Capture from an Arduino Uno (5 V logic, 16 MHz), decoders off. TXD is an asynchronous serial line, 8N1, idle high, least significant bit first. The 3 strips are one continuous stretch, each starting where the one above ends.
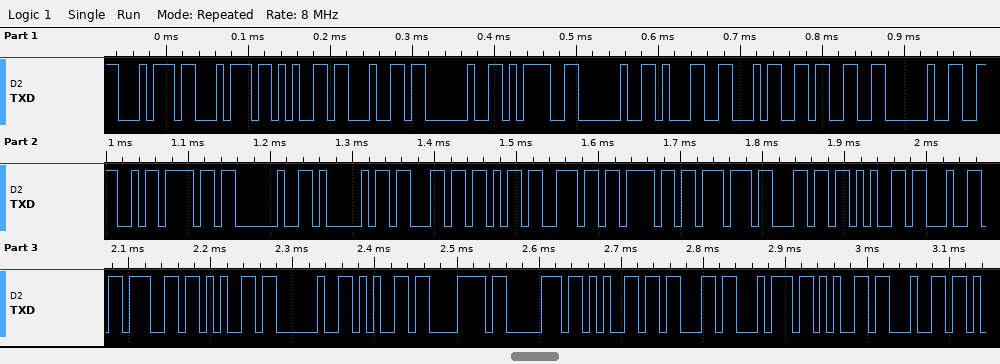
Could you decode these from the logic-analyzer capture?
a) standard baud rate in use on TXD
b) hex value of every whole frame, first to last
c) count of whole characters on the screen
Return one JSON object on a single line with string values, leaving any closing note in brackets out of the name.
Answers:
{"standard baud rate in use on TXD": "115200 baud", "hex value of every whole frame, first to last": "74 74 65 64 20 3D 20 31 34 33 20 4E 6F 20 41 63 6B 6E 6F 77 6C 65 64 67 65 20 65 78 70 65 63 74 65 64", "count of whole characters on the screen": "34"}
